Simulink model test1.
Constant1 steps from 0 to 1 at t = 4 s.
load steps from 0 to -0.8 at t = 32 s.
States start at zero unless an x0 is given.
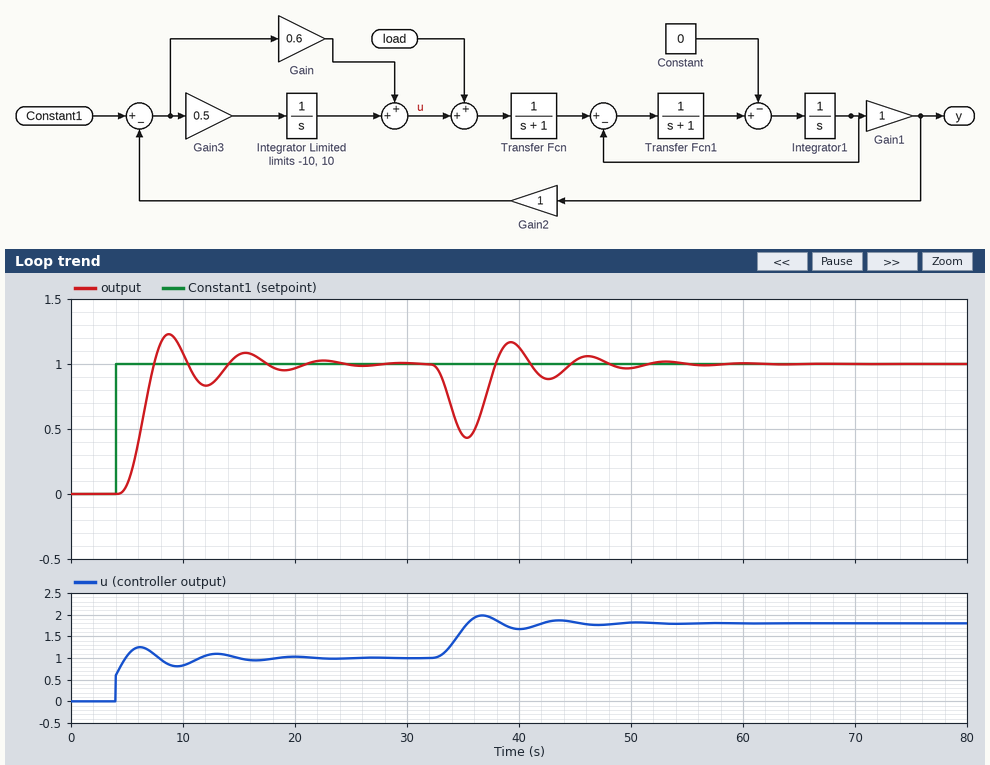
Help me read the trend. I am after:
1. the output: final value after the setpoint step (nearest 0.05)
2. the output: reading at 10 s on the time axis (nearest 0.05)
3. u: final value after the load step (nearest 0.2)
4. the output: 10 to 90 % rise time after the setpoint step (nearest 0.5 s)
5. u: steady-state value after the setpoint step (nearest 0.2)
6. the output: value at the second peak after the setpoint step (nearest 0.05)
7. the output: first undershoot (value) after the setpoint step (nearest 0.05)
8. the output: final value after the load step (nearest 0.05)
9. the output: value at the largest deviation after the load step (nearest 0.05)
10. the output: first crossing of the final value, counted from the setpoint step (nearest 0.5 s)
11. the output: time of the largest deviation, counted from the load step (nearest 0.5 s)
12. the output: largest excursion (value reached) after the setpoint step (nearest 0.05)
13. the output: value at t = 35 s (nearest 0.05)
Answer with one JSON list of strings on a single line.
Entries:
["1.00", "1.10", "1.8", "2.0 s", "1.0", "1.10", "0.85", "1.00", "0.45", "3.5 s", "3.5 s", "1.25", "0.45"]
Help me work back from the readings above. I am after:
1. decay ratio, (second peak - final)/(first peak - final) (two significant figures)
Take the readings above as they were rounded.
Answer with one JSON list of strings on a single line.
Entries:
["0.40"]
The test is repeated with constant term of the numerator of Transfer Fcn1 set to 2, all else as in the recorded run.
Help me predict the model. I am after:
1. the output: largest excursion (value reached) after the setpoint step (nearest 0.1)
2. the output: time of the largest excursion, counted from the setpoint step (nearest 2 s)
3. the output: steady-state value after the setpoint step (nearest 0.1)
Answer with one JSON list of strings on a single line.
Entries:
["1.1", "8 s", "1.0"]
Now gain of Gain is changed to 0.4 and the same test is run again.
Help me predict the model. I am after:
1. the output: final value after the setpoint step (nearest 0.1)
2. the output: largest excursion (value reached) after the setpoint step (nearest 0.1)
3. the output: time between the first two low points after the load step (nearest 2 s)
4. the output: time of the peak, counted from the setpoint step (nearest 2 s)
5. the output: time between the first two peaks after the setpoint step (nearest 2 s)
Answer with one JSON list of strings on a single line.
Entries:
["1.0", "1.3", "8 s", "6 s", "8 s"]
